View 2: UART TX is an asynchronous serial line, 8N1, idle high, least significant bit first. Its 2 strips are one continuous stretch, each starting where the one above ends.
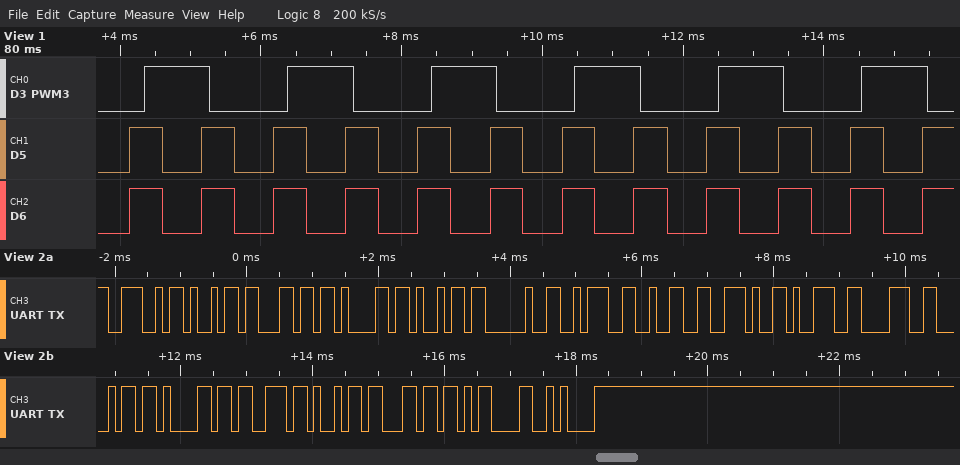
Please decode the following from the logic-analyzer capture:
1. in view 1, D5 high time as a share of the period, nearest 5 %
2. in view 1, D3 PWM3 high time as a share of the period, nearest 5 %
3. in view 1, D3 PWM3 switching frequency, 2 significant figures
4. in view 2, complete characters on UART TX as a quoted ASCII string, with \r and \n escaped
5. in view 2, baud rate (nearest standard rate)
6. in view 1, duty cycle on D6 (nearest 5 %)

45 %
45 %
490 Hz
"Nilai :2.98hasil\r\n"
9600 baud
45 %
